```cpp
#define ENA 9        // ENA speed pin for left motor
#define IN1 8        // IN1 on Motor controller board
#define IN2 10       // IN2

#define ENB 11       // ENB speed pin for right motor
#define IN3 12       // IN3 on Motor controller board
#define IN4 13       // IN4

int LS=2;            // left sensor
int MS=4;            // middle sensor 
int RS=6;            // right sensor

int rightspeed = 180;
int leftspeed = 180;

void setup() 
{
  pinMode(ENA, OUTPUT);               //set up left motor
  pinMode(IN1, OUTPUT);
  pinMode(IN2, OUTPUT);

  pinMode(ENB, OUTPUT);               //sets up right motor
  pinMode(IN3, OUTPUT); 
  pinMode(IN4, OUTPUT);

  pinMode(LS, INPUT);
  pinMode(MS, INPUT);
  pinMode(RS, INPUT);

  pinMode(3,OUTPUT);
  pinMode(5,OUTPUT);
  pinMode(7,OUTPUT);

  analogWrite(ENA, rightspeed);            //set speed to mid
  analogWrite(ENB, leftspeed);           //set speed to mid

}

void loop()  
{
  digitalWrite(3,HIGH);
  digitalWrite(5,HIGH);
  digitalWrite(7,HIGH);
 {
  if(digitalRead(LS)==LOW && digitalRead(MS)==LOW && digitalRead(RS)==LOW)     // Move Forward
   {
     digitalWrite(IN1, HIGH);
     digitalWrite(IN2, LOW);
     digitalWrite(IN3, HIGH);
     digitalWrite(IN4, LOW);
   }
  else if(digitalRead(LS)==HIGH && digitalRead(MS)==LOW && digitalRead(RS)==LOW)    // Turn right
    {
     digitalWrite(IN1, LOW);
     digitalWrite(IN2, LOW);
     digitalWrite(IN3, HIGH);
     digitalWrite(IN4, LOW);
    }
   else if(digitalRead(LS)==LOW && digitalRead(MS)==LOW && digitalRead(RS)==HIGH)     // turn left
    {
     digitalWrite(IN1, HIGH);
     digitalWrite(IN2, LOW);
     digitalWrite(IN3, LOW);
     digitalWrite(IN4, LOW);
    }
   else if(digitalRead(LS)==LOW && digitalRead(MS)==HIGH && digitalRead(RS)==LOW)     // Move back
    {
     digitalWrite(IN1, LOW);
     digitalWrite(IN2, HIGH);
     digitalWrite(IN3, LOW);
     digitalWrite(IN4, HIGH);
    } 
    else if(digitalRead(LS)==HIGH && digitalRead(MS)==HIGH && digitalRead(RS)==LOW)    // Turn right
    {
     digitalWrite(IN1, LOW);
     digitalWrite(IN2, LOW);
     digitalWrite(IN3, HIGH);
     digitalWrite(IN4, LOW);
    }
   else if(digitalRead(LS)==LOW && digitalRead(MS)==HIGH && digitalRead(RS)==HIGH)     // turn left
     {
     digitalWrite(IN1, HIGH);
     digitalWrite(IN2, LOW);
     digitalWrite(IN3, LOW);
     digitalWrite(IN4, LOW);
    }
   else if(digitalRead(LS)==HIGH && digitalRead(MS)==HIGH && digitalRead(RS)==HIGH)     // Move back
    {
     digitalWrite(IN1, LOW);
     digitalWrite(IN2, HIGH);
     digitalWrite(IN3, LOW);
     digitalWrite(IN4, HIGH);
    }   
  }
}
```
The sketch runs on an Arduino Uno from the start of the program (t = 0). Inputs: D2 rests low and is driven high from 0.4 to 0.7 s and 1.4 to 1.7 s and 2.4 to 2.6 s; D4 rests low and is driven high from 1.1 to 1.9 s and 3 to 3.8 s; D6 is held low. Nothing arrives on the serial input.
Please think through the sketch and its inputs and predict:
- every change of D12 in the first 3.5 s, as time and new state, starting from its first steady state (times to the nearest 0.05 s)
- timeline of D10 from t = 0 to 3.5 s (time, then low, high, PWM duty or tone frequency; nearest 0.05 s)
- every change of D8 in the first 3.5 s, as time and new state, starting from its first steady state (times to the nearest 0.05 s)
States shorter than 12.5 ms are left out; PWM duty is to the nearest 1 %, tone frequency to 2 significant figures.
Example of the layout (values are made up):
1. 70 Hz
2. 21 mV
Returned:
1. 0 s high; 1.1 s low; 1.4 s high; 1.7 s low; 1.9 s high; 3 s low
2. 0 s low; 1.1 s high; 1.4 s low; 1.7 s high; 1.9 s low; 3 s high
3. 0 s high; 0.4 s low; 0.7 s high; 1.1 s low; 1.9 s high; 2.4 s low; 2.6 s high; 3 s low
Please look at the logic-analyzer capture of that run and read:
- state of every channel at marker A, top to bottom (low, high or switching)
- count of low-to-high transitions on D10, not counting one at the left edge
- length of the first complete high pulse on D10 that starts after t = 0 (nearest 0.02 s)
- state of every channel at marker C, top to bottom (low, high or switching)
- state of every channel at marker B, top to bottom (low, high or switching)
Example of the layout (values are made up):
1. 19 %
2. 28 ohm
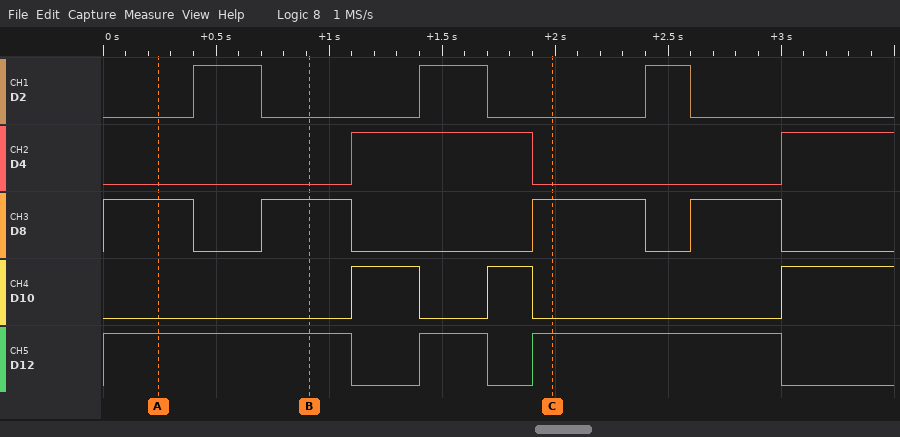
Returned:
1. D2 low, D4 low, D8 high, D10 low, D12 high
2. 3
3. 0.30 s
4. D2 low, D4 low, D8 high, D10 low, D12 high
5. D2 low, D4 low, D8 high, D10 low, D12 high
